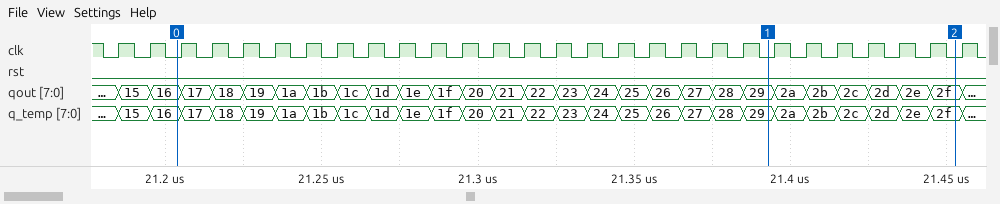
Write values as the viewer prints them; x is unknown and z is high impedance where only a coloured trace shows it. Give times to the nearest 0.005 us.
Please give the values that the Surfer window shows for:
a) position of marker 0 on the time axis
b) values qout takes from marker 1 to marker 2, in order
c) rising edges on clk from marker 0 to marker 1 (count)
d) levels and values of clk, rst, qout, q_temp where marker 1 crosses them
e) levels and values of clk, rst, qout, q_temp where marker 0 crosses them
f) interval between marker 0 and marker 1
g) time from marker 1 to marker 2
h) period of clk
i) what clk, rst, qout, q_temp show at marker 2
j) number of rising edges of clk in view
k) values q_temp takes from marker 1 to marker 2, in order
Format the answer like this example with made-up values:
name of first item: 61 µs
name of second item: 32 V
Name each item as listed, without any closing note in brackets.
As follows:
position of marker 0 on the time axis: 21.205 us
values qout takes from marker 1 to marker 2, in order: 29, 2a, 2b, 2c, 2d, 2e, 2f
rising edges on clk from marker 0 to marker 1: 19
levels and values of clk, rst, qout, q_temp where marker 1 crosses them: clk=0, rst=0, qout=29, q_temp=29
levels and values of clk, rst, qout, q_temp where marker 0 crosses them: clk=0, rst=0, qout=16, q_temp=16
interval between marker 0 and marker 1: 0.19 us
time from marker 1 to marker 2: 0.06 us
period of clk: 0.01 us
what clk, rst, qout, q_temp show at marker 2: clk=0, rst=0, qout=2f, q_temp=2f
number of rising edges of clk in view: 28
values q_temp takes from marker 1 to marker 2, in order: 29, 2a, 2b, 2c, 2d, 2e, 2f
